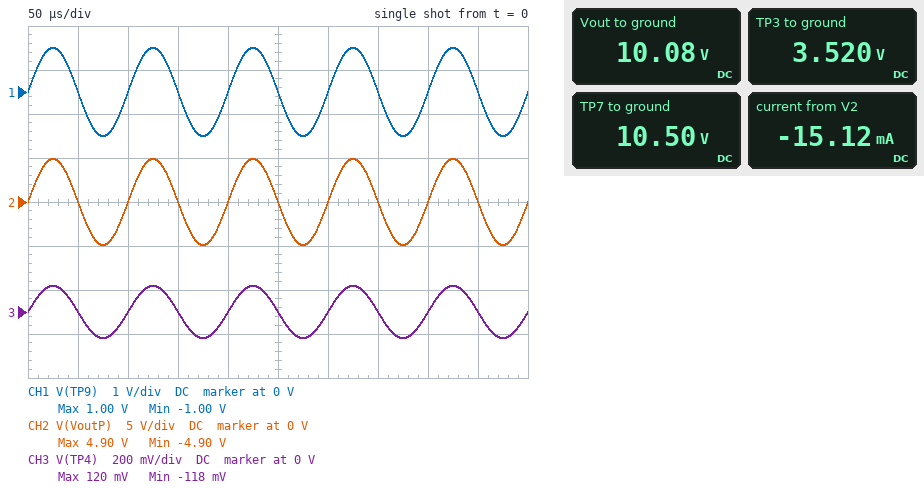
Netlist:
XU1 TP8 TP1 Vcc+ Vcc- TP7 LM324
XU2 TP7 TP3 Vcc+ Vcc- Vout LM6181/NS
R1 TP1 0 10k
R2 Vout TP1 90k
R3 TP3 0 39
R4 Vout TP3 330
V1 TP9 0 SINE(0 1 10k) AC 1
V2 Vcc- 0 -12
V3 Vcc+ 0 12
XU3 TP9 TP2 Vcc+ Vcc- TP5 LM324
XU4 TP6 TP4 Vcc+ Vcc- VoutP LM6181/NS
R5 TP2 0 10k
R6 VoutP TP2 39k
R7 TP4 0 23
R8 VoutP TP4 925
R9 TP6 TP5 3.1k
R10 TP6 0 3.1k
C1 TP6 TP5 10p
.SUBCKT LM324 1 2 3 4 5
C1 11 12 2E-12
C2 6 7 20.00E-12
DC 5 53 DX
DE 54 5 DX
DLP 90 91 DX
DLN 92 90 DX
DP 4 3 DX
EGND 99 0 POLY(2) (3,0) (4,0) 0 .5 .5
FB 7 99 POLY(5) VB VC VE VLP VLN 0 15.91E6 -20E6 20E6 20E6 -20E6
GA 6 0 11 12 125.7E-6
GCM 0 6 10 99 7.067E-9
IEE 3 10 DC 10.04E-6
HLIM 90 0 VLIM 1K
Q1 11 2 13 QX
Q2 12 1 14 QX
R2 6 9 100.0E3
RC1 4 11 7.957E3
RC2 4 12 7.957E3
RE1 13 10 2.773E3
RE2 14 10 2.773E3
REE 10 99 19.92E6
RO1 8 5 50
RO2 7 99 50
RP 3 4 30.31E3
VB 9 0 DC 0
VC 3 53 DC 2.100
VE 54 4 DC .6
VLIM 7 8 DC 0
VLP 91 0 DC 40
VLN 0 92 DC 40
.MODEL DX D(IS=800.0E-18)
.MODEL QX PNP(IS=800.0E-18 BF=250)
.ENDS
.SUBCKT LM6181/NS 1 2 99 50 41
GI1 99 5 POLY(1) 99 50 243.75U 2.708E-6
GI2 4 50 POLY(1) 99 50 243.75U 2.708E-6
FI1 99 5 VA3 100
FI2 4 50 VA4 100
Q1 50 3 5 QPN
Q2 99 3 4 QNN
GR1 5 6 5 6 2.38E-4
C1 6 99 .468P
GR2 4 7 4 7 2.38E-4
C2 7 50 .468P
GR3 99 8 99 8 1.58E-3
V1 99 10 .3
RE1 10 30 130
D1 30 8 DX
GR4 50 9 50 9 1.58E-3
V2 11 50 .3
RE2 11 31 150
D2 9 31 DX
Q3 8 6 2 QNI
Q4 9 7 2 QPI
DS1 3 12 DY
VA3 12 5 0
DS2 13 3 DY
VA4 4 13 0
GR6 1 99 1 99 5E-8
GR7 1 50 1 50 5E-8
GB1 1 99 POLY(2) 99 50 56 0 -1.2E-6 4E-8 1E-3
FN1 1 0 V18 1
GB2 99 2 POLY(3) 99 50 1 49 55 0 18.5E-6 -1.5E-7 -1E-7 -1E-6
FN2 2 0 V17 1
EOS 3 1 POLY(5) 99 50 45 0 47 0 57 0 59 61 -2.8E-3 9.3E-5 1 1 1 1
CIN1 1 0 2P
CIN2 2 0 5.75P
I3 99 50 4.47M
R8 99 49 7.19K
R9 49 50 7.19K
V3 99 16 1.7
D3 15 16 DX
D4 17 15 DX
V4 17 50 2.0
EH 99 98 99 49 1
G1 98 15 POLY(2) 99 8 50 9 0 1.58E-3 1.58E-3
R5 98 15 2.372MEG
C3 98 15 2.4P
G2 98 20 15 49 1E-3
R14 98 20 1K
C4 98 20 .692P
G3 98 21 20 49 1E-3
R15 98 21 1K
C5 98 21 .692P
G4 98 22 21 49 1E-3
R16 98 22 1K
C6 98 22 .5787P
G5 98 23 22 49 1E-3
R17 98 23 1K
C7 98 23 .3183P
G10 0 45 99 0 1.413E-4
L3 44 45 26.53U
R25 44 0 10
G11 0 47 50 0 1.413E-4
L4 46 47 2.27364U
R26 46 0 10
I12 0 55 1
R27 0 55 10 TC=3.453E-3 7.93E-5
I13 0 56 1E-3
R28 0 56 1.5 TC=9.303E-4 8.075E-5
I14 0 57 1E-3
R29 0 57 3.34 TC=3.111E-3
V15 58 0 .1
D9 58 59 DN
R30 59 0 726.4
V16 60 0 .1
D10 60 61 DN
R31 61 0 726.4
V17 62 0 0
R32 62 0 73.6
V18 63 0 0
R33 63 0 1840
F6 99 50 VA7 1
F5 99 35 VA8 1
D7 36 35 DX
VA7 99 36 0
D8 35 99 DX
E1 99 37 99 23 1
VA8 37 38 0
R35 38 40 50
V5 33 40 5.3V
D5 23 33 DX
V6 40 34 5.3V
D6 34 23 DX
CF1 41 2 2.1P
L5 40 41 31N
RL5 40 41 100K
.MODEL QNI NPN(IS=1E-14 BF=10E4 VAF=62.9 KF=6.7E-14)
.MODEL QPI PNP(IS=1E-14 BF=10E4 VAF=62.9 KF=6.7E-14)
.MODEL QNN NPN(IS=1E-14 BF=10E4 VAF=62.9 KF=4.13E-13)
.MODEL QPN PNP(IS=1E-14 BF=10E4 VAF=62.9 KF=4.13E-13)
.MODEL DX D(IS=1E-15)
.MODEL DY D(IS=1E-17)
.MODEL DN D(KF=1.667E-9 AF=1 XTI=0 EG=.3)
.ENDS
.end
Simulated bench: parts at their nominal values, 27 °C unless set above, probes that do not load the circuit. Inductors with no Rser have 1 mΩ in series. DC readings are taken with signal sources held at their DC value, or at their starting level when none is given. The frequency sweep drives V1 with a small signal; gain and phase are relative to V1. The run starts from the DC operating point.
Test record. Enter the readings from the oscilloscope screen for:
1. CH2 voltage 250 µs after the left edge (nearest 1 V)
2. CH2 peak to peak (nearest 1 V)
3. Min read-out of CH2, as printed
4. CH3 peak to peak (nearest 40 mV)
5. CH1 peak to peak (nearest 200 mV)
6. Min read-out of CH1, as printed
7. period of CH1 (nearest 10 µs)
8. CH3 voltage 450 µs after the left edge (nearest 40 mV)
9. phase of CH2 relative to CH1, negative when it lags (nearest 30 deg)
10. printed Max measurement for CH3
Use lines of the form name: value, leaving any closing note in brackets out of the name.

CH2 voltage 250 µs after the left edge: 0 V
CH2 peak to peak: 10 V
Min read-out of CH2, as printed: -4.90 V
CH3 peak to peak: 240 mV
CH1 peak to peak: 2.0 V
Min read-out of CH1, as printed: -1.00 V
period of CH1: 100 µs
CH3 voltage 450 µs after the left edge: 0 V
phase of CH2 relative to CH1, negative when it lags: 0 deg
printed Max measurement for CH3: 120 mV
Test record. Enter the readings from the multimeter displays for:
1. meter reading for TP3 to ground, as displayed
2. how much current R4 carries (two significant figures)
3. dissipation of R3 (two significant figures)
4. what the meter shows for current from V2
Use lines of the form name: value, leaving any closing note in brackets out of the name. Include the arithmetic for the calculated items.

meter reading for TP3 to ground, as displayed: 3.520 V
how much current R4 carries: (10.08 V - 3.52 V) / 330 Ω = 20 mA
dissipation of R3: (3.52 V)^2 / 39 Ω = 320 mW
what the meter shows for current from V2: -15.12 mA
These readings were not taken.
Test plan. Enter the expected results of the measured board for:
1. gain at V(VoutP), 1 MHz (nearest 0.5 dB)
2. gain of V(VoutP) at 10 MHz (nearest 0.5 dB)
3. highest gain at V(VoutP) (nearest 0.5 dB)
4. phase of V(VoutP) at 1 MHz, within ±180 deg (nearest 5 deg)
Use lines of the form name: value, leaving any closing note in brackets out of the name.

gain at V(VoutP), 1 MHz: 14.0 dB
gain of V(VoutP) at 10 MHz: 4.0 dB
highest gain at V(VoutP): 15.0 dB
phase of V(VoutP) at 1 MHz, within ±180 deg: -15 deg
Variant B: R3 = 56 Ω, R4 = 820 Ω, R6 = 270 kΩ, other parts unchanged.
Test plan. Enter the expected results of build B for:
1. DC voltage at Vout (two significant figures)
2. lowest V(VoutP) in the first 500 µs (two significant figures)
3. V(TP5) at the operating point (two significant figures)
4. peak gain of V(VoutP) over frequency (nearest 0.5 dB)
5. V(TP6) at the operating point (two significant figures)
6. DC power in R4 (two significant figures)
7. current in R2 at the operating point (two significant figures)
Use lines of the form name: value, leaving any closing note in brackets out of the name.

DC voltage at Vout: 11 V
lowest V(VoutP) in the first 500 µs: -10 V
V(TP5) at the operating point: -1.7 mV
peak gain of V(VoutP) over frequency: 29.0 dB
V(TP6) at the operating point: -2.8 mV
DC power in R4: 53 mW
current in R2 at the operating point: 110 µA
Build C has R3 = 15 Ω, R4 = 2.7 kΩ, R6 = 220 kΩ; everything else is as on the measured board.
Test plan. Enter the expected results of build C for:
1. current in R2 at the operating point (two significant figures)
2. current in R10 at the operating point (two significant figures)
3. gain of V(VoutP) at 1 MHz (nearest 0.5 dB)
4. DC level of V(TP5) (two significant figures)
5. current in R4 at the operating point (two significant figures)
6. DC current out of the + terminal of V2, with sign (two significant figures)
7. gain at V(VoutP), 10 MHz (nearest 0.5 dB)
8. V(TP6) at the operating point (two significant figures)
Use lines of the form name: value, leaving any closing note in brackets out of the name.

current in R2 at the operating point: 110 µA
current in R10 at the operating point: 900 nA
gain of V(VoutP) at 1 MHz: 24.5 dB
DC level of V(TP5): -1.7 mV
current in R4 at the operating point: 3.5 mA
DC current out of the + terminal of V2, with sign: -15 mA
gain at V(VoutP), 10 MHz: 2.0 dB
V(TP6) at the operating point: -2.8 mV
